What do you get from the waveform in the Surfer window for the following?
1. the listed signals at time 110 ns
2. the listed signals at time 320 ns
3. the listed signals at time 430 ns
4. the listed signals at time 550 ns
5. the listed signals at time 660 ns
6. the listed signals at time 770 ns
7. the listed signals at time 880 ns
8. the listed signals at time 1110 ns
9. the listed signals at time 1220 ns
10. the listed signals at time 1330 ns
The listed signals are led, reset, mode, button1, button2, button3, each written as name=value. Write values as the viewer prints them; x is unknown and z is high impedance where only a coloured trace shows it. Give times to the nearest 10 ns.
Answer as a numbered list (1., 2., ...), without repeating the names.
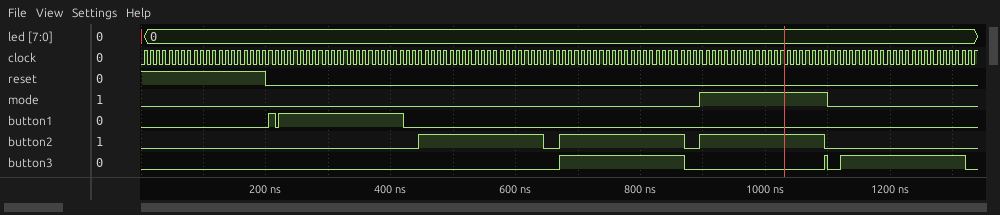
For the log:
1. led=0, reset=1, mode=0, button1=0, button2=0, button3=0
2. led=0, reset=0, mode=0, button1=1, button2=0, button3=0
3. led=0, reset=0, mode=0, button1=0, button2=0, button3=0
4. led=0, reset=0, mode=0, button1=0, button2=1, button3=0
5. led=0, reset=0, mode=0, button1=0, button2=0, button3=0
6. led=0, reset=0, mode=0, button1=0, button2=1, button3=1
7. led=0, reset=0, mode=0, button1=0, button2=0, button3=0
8. led=0, reset=0, mode=0, button1=0, button2=0, button3=0
9. led=0, reset=0, mode=0, button1=0, button2=0, button3=1
10. led=0, reset=0, mode=0, button1=0, button2=0, button3=0
